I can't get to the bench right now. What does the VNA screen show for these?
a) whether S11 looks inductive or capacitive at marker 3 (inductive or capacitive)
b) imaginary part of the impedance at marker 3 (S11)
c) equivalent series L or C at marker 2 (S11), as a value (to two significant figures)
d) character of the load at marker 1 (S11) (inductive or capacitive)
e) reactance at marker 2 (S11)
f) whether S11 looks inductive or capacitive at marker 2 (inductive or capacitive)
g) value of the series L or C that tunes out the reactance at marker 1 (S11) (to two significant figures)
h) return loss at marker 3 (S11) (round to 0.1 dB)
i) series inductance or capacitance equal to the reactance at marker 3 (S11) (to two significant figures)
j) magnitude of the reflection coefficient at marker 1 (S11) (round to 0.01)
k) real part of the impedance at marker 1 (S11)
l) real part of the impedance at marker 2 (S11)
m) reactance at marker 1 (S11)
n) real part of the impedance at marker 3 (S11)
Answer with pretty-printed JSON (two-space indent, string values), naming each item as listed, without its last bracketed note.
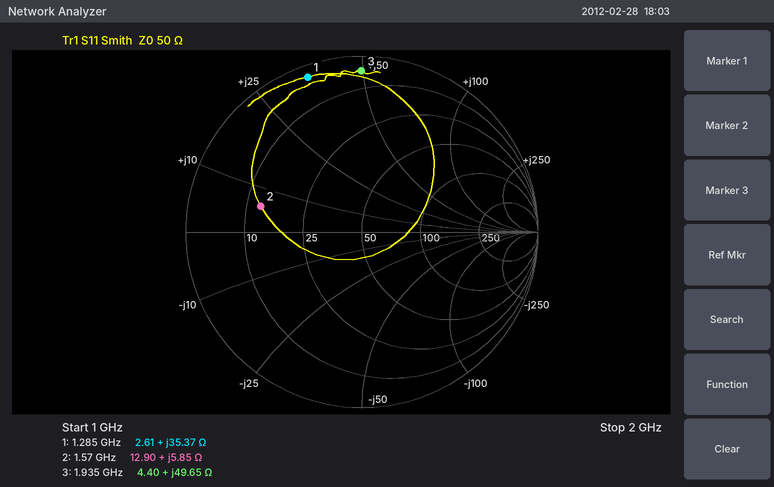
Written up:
{
  "whether S11 looks inductive or capacitive at marker 3": "inductive",
  "imaginary part of the impedance at marker 3": "+49.65 Ω",
  "equivalent series L or C at marker 2 (S11), as a value": "590 pH",
  "character of the load at marker 1 (S11)": "inductive",
  "reactance at marker 2": "+5.85 Ω",
  "whether S11 looks inductive or capacitive at marker 2": "inductive",
  "value of the series L or C that tunes out the reactance at marker 1 (S11)": "3.5 pF",
  "return loss at marker 3 (S11)": "0.8 dB",
  "series inductance or capacitance equal to the reactance at marker 3 (S11)": "4.1 nH",
  "magnitude of the reflection coefficient at marker 1 (S11)": "0.93",
  "real part of the impedance at marker 1": "2.61 Ω",
  "real part of the impedance at marker 2": "12.90 Ω",
  "reactance at marker 1": "+35.37 Ω",
  "real part of the impedance at marker 3": "4.40 Ω"
}
